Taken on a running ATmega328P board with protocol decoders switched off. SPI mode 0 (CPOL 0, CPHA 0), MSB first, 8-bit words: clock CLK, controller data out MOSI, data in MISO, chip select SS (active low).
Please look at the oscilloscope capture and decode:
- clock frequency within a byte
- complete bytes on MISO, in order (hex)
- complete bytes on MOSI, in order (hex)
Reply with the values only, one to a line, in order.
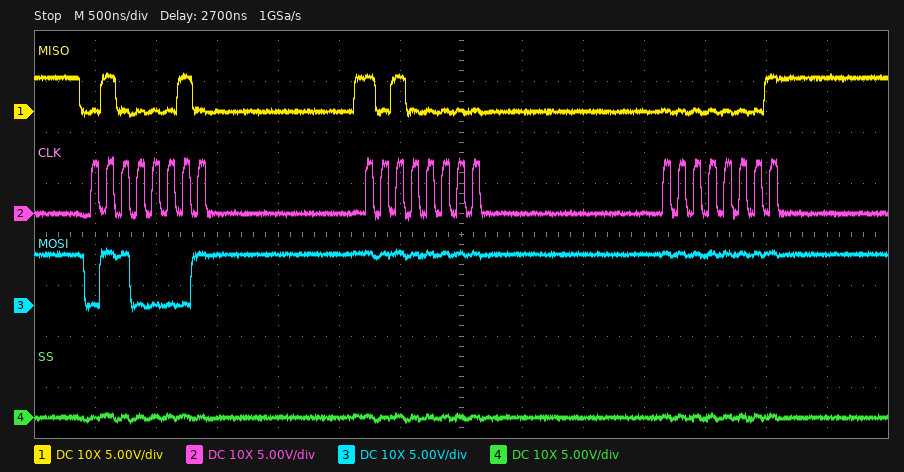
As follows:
8 MHz
42 A0 01
61 FF FF
